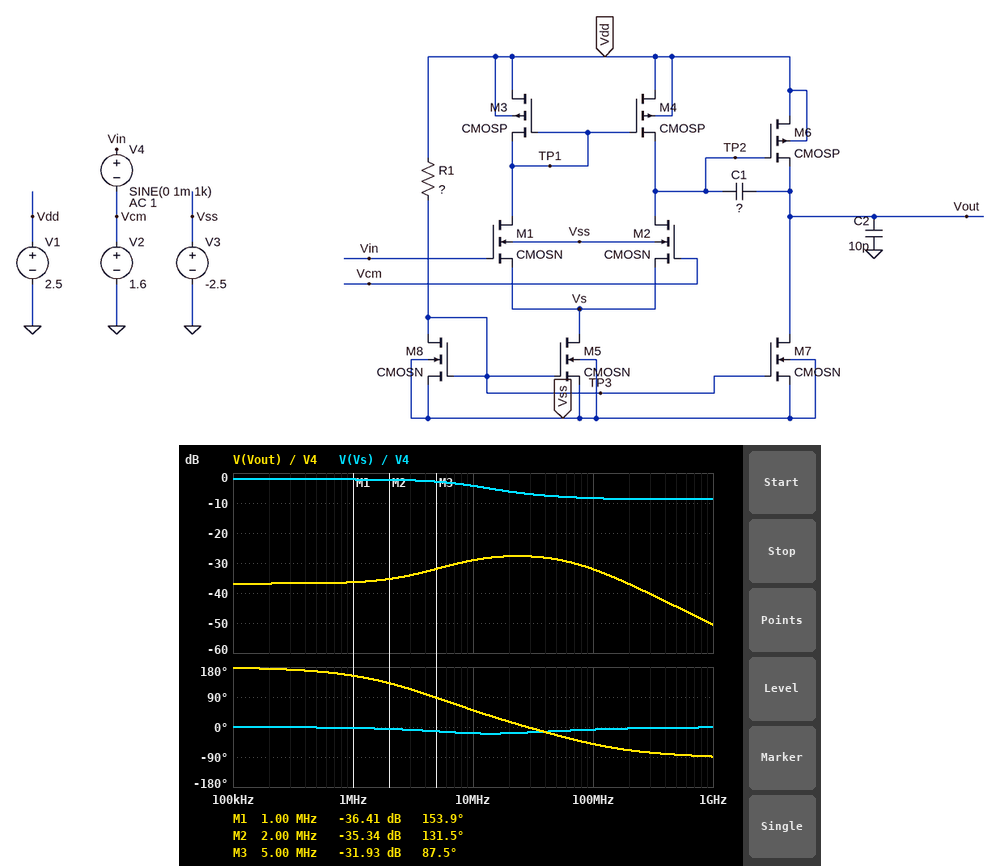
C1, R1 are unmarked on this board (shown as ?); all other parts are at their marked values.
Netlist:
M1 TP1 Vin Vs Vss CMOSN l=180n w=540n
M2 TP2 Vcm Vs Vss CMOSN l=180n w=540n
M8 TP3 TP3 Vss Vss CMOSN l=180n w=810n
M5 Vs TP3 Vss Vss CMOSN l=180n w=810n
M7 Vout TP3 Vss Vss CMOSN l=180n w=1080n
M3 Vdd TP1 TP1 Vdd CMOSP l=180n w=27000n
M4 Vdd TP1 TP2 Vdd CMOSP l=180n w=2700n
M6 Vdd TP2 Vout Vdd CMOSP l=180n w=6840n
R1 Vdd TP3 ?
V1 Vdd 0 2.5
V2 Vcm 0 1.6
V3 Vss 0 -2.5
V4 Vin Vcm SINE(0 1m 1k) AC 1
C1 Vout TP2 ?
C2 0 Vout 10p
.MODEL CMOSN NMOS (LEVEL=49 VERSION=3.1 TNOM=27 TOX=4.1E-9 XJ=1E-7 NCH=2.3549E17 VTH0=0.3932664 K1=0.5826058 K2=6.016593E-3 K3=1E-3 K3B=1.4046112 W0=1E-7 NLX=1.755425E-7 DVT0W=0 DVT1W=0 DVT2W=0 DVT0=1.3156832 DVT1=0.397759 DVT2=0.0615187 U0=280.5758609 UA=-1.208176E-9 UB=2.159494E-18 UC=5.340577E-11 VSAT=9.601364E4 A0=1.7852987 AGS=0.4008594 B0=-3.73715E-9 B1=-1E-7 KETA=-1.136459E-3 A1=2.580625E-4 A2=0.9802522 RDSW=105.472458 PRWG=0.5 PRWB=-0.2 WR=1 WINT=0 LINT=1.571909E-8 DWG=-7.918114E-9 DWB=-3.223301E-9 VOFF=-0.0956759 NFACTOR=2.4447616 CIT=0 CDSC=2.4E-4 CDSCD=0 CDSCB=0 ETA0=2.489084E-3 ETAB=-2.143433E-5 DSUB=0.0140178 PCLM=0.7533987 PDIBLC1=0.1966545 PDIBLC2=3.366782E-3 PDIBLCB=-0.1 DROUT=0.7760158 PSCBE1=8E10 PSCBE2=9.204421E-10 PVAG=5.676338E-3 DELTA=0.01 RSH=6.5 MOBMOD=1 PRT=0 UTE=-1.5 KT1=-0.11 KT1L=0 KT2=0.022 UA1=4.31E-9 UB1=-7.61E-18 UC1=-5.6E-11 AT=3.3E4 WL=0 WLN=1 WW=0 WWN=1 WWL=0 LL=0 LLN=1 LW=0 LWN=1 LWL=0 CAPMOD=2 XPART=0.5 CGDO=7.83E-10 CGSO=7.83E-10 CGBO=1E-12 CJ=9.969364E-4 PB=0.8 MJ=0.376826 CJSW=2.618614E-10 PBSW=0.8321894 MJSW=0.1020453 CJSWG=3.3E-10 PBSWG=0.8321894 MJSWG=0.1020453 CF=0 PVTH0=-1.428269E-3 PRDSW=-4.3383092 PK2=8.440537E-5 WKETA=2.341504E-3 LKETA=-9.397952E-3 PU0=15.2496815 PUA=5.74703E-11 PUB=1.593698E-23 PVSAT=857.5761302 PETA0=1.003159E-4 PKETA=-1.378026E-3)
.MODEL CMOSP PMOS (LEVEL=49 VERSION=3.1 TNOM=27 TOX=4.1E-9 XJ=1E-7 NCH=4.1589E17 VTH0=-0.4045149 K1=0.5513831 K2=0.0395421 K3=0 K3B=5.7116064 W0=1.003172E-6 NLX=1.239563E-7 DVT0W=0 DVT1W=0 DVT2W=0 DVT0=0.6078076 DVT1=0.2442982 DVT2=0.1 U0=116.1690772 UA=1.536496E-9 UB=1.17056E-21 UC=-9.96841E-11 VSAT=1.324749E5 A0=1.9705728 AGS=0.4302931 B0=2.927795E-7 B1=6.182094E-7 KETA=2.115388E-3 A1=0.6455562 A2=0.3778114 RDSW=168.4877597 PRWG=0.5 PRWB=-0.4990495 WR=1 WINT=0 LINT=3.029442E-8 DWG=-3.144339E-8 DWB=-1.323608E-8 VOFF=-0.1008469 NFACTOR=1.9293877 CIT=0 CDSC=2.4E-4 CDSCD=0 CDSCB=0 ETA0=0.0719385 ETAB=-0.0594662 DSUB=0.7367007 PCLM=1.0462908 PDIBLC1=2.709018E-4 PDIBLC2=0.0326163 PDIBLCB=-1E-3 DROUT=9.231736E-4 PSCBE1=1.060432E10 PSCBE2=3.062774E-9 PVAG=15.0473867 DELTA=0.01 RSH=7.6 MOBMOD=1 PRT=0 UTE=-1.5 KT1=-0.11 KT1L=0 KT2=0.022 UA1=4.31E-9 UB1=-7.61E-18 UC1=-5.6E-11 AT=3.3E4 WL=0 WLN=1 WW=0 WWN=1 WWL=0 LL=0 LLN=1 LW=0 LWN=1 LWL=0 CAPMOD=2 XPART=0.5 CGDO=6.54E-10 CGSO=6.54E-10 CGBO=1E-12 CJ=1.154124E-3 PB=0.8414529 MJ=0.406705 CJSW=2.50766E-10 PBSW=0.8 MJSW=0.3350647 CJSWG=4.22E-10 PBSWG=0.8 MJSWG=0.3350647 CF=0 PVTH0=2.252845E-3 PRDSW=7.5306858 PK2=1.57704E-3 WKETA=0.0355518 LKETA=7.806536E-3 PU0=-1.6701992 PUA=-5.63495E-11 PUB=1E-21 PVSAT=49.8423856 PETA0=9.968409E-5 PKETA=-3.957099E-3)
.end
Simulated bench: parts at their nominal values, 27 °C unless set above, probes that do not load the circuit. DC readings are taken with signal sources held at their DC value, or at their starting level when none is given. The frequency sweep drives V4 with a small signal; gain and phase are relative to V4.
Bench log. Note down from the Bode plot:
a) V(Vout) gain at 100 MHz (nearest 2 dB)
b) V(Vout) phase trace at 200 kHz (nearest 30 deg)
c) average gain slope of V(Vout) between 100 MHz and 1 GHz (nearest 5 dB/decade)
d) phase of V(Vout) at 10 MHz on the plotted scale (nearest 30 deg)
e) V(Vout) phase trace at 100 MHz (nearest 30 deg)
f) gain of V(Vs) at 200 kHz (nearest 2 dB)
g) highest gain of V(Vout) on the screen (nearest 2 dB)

-32 dB
180 deg
-20 dB/decade
60 deg
-60 deg
-2 dB
-28 dB
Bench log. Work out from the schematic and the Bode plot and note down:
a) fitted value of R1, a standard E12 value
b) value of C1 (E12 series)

33 kΩ
3.3 pF
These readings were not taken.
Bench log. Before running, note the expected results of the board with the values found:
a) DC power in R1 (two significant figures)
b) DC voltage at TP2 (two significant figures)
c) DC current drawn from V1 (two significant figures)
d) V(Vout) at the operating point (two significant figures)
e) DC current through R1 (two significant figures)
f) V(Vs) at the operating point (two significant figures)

500 µW
140 mV
510 µA
2.4 V
120 µA
80 mV
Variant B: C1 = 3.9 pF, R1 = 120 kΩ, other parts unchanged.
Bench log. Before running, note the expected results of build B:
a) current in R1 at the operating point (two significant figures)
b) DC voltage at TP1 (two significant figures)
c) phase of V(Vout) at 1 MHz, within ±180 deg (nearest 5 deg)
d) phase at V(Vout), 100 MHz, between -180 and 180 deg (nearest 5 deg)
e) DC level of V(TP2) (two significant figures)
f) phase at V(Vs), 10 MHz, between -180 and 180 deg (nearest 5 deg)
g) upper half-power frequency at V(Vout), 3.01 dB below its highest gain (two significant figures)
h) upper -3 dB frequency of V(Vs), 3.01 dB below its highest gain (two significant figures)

36 µA
1.9 V
130 deg
-55 deg
370 mV
-15 deg
67 MHz
8.7 MHz
